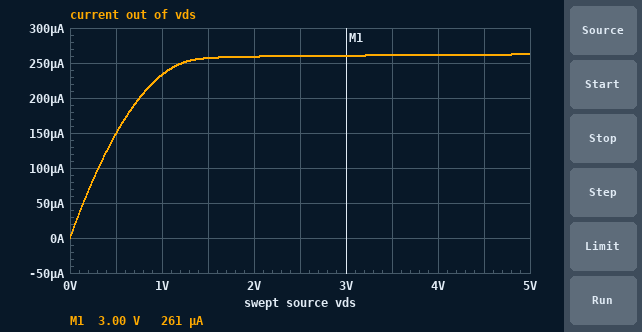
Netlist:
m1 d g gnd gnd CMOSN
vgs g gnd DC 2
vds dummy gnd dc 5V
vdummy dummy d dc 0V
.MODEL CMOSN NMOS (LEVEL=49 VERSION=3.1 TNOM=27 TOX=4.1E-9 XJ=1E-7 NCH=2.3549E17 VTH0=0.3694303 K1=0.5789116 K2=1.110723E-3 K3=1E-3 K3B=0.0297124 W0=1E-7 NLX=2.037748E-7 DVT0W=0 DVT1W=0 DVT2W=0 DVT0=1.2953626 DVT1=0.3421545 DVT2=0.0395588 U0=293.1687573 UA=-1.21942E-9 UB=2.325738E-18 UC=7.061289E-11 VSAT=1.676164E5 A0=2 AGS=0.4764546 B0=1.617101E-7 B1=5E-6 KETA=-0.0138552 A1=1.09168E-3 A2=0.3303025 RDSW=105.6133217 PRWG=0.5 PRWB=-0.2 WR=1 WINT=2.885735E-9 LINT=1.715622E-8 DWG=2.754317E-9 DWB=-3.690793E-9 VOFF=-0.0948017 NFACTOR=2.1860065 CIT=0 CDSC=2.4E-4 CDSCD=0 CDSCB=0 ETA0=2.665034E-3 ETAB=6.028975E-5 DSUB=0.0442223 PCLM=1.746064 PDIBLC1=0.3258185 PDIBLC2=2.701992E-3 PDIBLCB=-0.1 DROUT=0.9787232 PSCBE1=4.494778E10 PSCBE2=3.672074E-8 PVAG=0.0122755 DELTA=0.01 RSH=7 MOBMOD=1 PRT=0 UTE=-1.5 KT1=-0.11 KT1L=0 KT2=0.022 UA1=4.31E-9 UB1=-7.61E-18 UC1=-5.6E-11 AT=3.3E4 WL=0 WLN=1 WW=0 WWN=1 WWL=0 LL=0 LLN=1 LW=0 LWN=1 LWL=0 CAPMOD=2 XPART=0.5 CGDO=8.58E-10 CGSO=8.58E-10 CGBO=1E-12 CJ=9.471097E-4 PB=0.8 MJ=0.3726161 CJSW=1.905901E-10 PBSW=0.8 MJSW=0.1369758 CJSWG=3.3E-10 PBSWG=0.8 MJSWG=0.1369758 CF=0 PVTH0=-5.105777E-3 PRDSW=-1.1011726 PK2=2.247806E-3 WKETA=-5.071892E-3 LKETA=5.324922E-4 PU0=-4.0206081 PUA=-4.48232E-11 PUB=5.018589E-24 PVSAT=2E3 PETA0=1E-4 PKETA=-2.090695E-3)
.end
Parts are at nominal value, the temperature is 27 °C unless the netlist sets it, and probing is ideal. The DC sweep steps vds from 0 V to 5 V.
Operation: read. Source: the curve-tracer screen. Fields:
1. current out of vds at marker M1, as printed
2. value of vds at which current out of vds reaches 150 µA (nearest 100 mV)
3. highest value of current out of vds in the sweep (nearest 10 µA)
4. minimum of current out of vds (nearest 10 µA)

261 µA
500 mV
260 µA
0 A
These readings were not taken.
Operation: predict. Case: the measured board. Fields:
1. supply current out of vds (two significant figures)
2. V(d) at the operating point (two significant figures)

260 µA
5.0 V
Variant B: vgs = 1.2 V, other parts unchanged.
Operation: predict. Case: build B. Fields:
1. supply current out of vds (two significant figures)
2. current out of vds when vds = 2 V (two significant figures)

74 µA
73 µA
